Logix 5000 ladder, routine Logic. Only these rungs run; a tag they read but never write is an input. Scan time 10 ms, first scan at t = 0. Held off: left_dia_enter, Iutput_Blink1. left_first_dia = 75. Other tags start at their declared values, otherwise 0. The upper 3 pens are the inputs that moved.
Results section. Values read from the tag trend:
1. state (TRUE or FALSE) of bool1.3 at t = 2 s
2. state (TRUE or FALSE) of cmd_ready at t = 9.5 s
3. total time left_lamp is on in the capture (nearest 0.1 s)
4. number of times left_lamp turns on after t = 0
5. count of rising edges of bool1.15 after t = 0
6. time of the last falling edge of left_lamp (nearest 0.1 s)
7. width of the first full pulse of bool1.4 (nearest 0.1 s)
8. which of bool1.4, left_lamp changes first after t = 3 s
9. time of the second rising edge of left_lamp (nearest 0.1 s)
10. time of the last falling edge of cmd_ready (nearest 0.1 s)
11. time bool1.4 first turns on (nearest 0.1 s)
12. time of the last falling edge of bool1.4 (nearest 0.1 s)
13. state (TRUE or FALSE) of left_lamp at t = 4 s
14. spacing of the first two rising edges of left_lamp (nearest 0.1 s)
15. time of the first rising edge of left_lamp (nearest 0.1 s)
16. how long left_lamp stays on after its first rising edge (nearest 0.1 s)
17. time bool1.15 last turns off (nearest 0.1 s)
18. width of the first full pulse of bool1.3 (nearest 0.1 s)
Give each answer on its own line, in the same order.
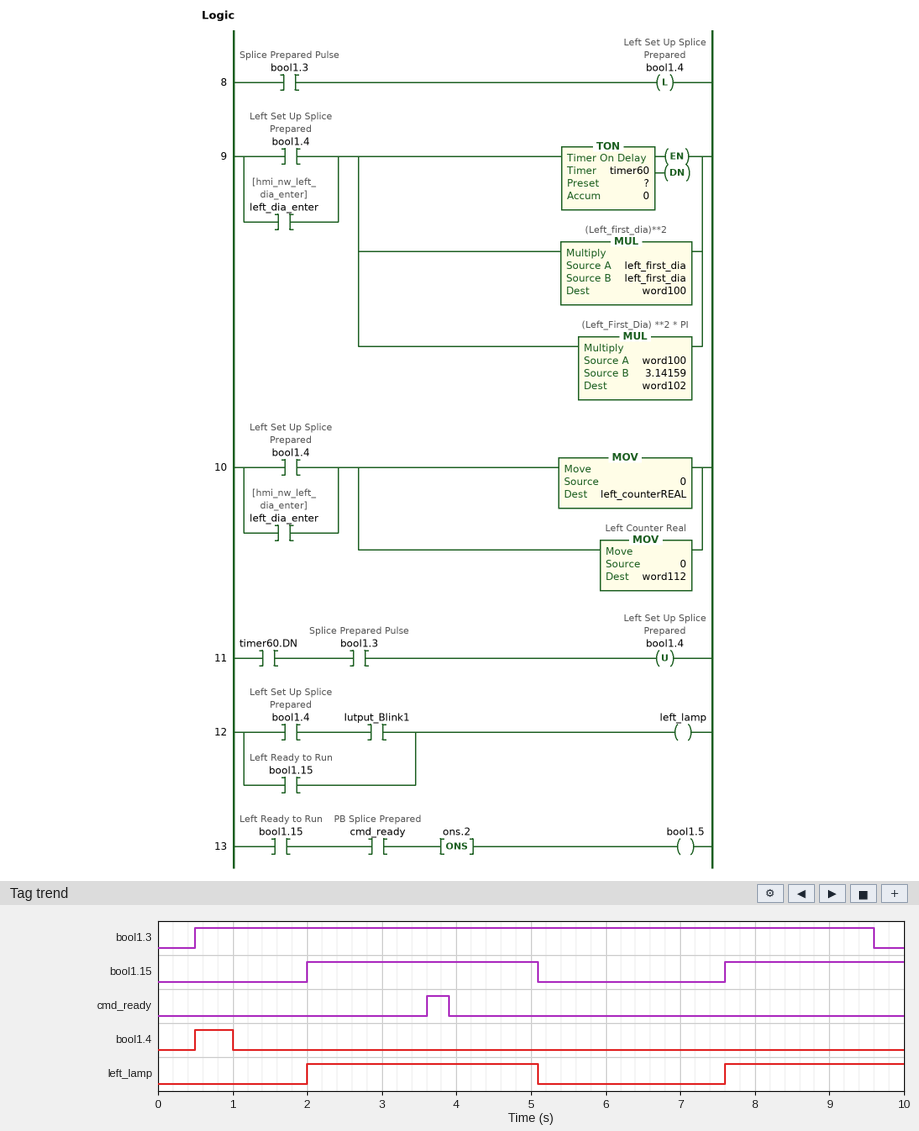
TRUE
FALSE
5.5 s
2
2
5.1 s
0.5 s
left_lamp
7.6 s
3.9 s
0.5 s
1.0 s
TRUE
5.6 s
2.0 s
3.1 s
5.1 s
9.1 s
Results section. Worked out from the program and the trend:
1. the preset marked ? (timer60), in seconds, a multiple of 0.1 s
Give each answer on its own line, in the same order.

0.5 s
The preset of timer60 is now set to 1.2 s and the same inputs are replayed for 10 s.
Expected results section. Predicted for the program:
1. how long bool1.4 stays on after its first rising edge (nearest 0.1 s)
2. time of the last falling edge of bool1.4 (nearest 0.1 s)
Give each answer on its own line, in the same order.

1.2 s
1.7 s
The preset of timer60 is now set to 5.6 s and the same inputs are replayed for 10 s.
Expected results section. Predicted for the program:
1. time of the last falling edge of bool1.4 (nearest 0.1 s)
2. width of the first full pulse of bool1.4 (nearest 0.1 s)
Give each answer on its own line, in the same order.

6.1 s
5.6 s
